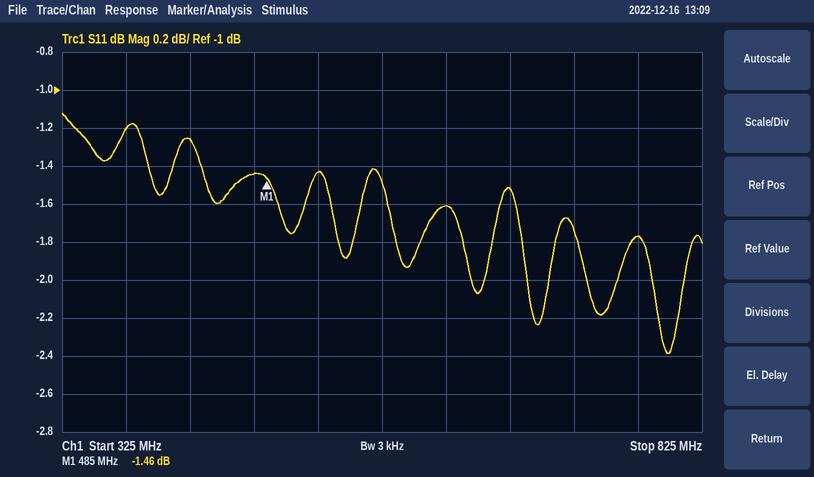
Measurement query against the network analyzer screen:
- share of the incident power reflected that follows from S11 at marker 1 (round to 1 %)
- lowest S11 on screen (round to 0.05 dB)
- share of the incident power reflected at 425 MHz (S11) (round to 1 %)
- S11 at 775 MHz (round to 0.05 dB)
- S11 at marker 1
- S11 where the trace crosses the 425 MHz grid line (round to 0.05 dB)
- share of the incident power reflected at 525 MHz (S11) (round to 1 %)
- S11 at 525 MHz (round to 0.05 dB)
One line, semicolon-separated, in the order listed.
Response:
71 %; -2.40 dB; 75 %; -1.75 dB; -1.46 dB; -1.25 dB; 72 %; -1.45 dB
